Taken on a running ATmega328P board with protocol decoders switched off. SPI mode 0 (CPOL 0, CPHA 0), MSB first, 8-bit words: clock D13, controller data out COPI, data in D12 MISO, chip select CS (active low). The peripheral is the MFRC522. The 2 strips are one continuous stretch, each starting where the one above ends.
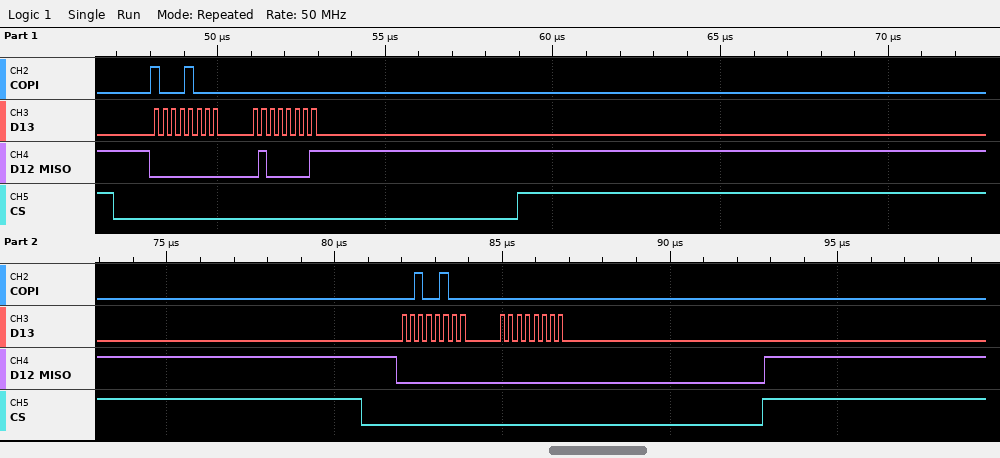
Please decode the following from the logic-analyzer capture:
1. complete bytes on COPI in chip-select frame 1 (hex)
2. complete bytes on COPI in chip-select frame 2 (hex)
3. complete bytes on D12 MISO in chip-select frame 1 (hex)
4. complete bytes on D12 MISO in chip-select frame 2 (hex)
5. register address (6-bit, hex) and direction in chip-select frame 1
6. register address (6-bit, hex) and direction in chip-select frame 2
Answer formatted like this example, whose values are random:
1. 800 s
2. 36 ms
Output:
1. 0x88 0x00
2. 0x24 0x00
3. 0x00 0x41
4. 0x00 0x00
5. 0x04 read
6. 0x12 write
